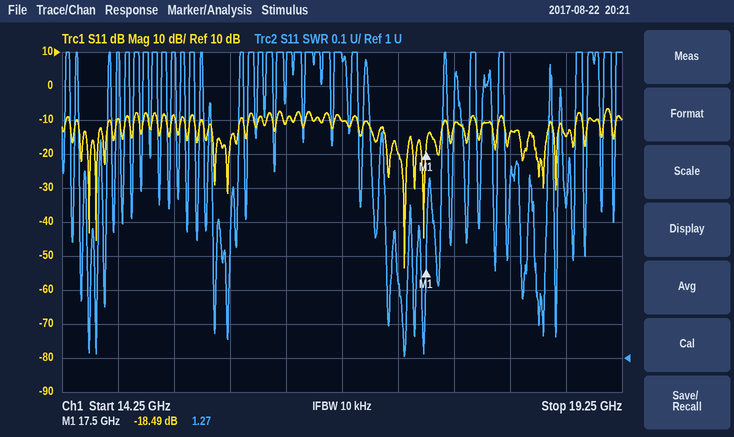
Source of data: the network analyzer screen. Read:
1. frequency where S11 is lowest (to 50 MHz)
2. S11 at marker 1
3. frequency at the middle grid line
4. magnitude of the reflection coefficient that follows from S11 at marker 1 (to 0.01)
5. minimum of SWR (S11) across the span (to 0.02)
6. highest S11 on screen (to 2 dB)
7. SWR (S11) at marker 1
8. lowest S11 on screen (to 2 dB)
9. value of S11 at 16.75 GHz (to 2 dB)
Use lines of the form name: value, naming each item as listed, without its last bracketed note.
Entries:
frequency where S11 is lowest: 17.30 GHz
S11 at marker 1: -18.49 dB
frequency at the middle grid line: 16.75 GHz
magnitude of the reflection coefficient that follows from S11 at marker 1: 0.12
minimum of SWR (S11) across the span: 1.00
highest S11 on screen: -6 dB
SWR (S11) at marker 1: 1.27
lowest S11 on screen: -54 dB
value of S11 at 16.75 GHz: -10 dB
